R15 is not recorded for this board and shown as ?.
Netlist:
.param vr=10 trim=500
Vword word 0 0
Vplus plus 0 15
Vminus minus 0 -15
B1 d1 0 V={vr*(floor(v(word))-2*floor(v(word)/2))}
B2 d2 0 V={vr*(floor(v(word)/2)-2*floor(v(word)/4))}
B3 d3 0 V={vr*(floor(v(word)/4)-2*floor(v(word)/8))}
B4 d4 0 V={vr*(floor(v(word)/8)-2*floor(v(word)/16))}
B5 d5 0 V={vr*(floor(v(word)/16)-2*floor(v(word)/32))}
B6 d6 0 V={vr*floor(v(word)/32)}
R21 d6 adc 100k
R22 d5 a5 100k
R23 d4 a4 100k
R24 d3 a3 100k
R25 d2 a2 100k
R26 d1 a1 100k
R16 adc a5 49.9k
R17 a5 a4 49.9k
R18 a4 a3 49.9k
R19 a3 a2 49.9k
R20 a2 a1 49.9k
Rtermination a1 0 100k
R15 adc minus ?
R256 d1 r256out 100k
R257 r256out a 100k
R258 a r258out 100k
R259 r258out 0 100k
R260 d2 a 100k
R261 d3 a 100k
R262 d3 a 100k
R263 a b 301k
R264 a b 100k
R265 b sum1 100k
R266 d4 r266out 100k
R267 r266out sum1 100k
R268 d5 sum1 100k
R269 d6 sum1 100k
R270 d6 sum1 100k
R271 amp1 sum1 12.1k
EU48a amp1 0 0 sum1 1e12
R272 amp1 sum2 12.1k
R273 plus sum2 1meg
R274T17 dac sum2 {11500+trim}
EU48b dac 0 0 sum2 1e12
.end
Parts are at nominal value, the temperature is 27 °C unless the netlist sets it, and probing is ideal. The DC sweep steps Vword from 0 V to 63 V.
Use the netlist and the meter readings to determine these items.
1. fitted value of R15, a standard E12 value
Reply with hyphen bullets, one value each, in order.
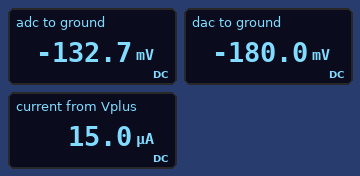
- 5.6 MΩ
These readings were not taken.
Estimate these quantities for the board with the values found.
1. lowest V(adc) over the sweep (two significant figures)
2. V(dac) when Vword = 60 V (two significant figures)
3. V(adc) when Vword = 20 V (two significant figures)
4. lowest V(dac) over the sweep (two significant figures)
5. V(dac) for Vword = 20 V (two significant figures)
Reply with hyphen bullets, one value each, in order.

- -130 mV
- 4.3 V
- 3.0 V
- -180 mV
- 1.3 V
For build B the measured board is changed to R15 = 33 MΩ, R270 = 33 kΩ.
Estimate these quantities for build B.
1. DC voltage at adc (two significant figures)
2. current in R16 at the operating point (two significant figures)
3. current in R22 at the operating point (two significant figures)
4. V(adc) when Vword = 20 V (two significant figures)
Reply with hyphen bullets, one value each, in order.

- -23 mV
- 230 nA
- 110 nA
- 3.1 V
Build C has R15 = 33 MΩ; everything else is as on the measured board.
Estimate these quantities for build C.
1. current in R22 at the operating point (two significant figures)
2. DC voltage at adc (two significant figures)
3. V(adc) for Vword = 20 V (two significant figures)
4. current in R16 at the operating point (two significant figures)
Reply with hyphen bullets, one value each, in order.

- 110 nA
- -23 mV
- 3.1 V
- 230 nA
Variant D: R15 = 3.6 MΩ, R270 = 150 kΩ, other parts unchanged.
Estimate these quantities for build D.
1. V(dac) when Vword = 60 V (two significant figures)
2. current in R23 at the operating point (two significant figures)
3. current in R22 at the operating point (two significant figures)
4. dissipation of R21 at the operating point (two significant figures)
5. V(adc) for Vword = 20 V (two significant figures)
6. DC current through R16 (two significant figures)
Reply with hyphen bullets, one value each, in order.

- 3.9 V
- 510 nA
- 1.0 µA
- 420 nW
- 2.9 V
- 2.1 µA
